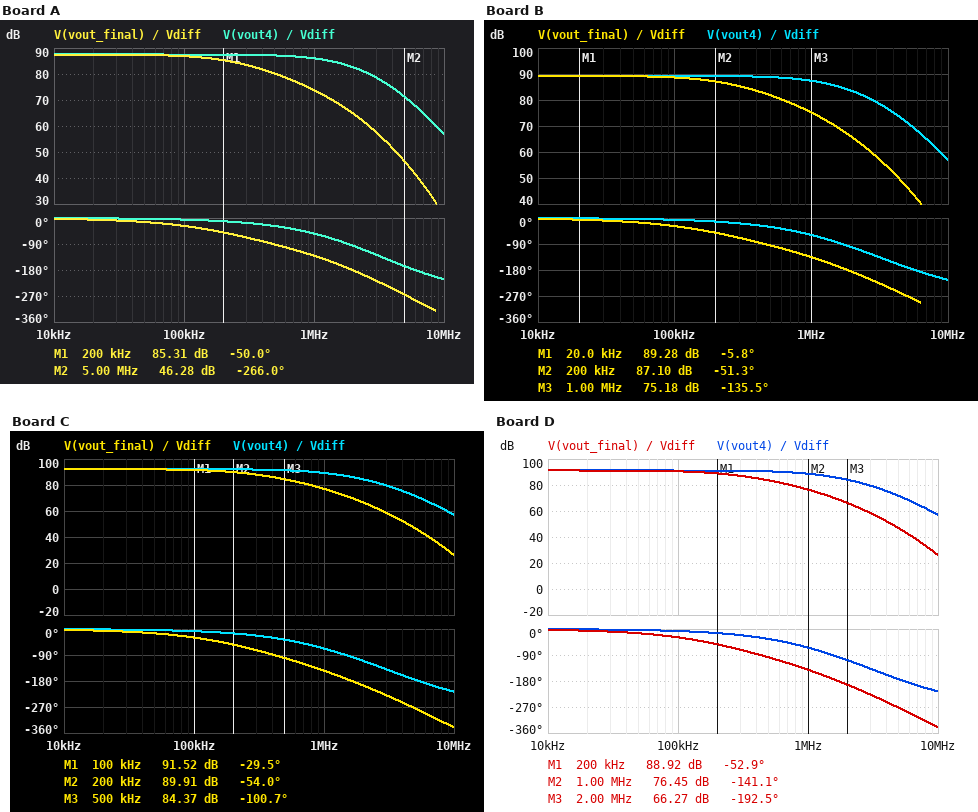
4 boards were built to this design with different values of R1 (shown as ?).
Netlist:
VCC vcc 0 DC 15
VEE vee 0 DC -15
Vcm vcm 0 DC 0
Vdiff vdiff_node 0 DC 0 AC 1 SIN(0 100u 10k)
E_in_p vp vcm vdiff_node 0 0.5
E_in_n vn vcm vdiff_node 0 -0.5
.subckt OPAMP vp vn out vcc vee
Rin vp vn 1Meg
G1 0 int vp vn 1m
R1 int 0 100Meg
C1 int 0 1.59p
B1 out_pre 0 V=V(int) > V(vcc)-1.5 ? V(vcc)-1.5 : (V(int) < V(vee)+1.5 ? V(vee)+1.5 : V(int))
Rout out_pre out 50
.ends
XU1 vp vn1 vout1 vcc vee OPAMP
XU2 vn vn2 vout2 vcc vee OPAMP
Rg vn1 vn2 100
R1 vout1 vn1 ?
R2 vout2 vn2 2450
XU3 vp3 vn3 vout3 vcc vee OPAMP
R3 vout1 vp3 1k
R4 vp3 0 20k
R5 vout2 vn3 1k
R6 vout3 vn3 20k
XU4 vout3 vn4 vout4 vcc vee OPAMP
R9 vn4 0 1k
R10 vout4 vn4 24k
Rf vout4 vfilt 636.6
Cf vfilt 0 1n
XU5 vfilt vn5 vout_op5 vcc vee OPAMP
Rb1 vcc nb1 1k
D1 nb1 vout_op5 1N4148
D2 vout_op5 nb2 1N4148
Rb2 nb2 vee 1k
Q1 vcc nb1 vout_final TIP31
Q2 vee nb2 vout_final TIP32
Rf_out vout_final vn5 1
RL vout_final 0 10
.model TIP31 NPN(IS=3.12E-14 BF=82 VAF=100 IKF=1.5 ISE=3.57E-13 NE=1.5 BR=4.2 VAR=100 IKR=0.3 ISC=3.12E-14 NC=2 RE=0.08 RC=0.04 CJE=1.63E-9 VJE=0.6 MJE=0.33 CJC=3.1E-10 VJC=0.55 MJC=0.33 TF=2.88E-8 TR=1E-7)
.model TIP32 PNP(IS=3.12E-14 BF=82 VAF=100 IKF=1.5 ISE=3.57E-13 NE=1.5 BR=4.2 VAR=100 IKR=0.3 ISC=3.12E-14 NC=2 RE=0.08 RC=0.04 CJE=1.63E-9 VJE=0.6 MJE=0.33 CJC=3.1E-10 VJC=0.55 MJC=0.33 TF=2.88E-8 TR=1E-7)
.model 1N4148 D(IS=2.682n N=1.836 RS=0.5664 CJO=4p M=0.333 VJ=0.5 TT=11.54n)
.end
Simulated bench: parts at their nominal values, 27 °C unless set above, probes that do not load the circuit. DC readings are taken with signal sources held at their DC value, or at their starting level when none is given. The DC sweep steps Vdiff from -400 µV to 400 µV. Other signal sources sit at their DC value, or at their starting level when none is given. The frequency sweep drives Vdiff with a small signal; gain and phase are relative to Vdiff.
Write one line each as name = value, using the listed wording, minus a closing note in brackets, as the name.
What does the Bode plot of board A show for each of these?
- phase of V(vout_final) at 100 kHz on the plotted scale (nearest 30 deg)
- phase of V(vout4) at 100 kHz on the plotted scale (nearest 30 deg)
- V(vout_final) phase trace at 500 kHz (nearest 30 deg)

phase of V(vout_final) at 100 kHz on the plotted scale = -30 deg
phase of V(vout4) at 100 kHz on the plotted scale = 0 deg
V(vout_final) phase trace at 500 kHz = -90 deg
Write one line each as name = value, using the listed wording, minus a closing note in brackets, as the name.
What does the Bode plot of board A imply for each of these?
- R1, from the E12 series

R1, from the E12 series = 2.2 kΩ
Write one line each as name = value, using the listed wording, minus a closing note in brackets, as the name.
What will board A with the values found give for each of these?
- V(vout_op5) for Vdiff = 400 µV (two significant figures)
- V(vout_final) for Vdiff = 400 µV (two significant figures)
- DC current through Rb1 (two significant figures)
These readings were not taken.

V(vout_op5) for Vdiff = 400 µV = 12 V
V(vout_final) for Vdiff = 400 µV = 5.6 V
DC current through Rb1 = 14 mA
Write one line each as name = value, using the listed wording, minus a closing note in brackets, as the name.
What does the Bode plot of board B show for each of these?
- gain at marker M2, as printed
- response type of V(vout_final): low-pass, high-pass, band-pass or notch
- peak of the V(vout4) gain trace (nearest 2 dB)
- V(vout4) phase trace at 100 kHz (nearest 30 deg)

gain at marker M2, as printed = 87.10 dB
response type of V(vout_final): low-pass, high-pass, band-pass or notch = low-pass
peak of the V(vout4) gain trace = 90 dB
V(vout4) phase trace at 100 kHz = 0 deg
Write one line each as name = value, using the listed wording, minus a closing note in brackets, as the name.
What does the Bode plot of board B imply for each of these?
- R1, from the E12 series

R1, from the E12 series = 3.3 kΩ
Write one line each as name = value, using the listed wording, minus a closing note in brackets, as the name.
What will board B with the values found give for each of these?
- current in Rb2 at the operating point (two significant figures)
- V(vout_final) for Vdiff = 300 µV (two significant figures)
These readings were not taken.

current in Rb2 at the operating point = 14 mA
V(vout_final) for Vdiff = 300 µV = 5.6 V
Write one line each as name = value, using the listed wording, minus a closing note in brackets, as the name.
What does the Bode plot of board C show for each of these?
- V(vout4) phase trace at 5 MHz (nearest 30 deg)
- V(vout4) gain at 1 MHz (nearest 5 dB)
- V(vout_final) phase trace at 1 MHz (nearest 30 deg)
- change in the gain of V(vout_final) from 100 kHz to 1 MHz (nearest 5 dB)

V(vout4) phase trace at 5 MHz = -180 deg
V(vout4) gain at 1 MHz = 90 dB
V(vout_final) phase trace at 1 MHz = -150 deg
change in the gain of V(vout_final) from 100 kHz to 1 MHz = -15 dB
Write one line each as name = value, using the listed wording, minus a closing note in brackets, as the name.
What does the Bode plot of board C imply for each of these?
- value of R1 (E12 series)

value of R1 = 5.6 kΩ
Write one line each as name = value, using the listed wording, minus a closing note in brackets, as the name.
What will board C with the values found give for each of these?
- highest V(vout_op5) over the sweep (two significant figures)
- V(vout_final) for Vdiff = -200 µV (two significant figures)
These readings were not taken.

highest V(vout_op5) over the sweep = 12 V
V(vout_final) for Vdiff = -200 µV = -5.6 V
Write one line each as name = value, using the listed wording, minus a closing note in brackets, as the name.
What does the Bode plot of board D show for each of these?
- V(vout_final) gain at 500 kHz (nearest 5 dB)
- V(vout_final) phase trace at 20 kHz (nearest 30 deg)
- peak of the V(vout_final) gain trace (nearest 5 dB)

V(vout_final) gain at 500 kHz = 85 dB
V(vout_final) phase trace at 20 kHz = 0 deg
peak of the V(vout_final) gain trace = 90 dB
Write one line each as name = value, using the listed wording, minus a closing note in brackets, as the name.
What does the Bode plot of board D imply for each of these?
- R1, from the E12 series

R1, from the E12 series = 4.7 kΩ
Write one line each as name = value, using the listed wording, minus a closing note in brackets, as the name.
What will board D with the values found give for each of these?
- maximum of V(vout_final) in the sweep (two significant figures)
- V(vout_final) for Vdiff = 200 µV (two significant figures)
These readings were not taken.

maximum of V(vout_final) in the sweep = 5.6 V
V(vout_final) for Vdiff = 200 µV = 5.6 V
